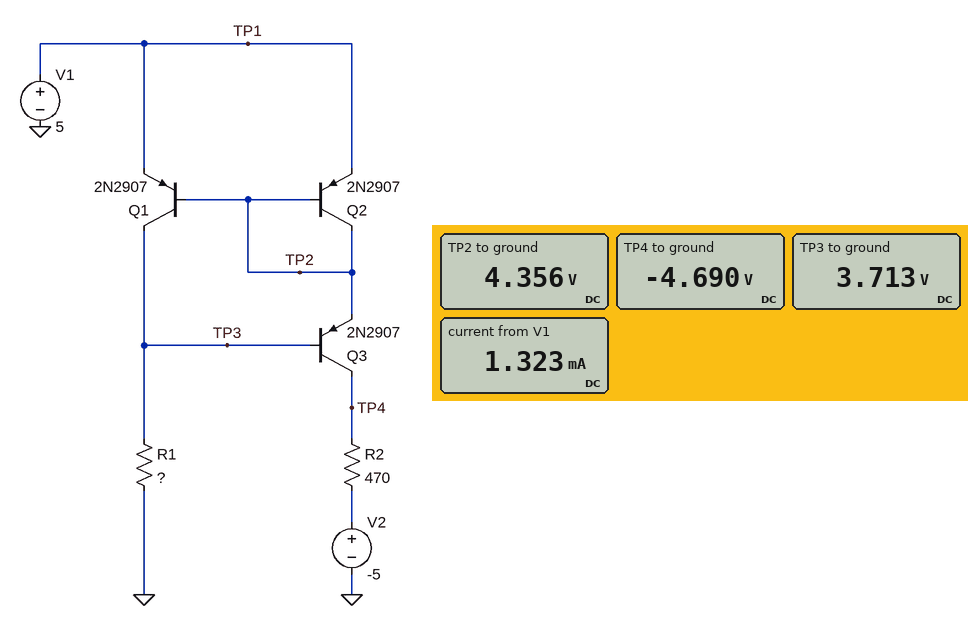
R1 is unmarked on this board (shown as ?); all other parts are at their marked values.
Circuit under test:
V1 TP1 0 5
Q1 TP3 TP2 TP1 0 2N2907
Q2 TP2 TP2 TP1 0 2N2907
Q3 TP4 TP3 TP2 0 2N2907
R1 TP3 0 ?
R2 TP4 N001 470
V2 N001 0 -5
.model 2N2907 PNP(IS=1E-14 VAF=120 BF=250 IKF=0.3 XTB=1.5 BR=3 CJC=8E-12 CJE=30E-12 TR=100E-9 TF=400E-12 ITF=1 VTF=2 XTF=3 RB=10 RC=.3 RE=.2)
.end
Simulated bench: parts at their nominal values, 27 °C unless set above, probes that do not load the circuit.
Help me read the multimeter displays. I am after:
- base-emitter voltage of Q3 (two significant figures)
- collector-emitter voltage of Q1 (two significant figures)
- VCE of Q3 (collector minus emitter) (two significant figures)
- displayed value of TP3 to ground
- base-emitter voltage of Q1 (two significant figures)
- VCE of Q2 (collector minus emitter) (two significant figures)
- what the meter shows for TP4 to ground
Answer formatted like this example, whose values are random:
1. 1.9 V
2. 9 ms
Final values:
1. -640 mV
2. -1.3 V
3. -9.0 V
4. 3.713 V
5. -640 mV
6. -640 mV
7. -4.690 V
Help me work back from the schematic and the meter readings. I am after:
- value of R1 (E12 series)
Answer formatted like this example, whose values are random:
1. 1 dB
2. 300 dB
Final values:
1. 5.6 kΩ
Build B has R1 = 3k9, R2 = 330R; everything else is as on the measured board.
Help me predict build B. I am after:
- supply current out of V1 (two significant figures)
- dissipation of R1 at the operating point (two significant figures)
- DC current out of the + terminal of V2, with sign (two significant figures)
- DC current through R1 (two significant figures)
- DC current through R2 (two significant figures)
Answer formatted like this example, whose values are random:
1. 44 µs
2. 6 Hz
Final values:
1. 1.9 mA
2. 3.5 mW
3. -940 µA
4. 950 µA
5. 940 µA
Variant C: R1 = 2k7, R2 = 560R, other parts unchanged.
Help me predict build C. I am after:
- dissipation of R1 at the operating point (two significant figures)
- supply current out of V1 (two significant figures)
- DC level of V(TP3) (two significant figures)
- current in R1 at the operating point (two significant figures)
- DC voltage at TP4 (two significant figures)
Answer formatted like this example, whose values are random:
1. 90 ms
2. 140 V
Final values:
1. 5.0 mW
2. 2.7 mA
3. 3.7 V
4. 1.4 mA
5. -4.2 V
